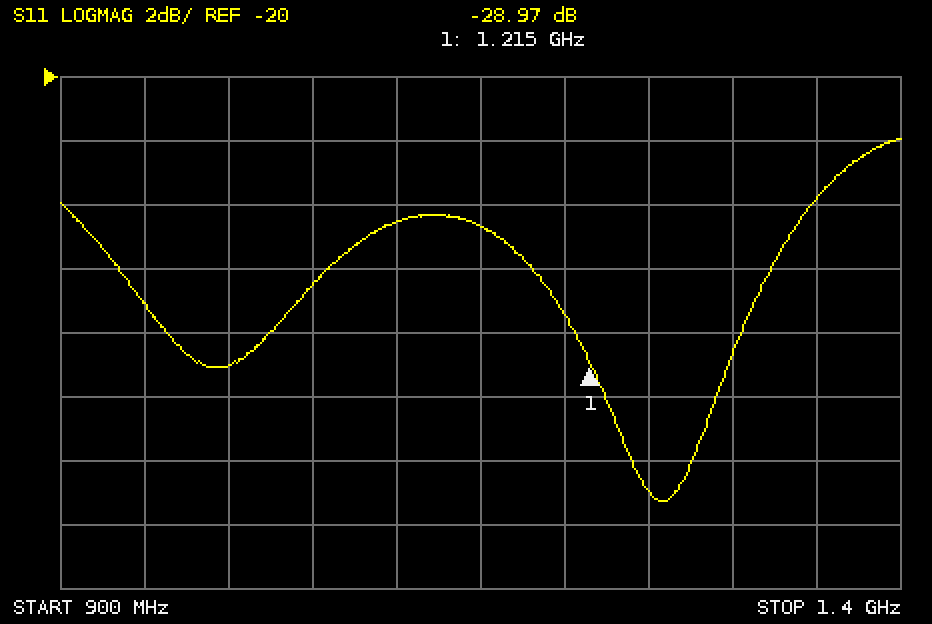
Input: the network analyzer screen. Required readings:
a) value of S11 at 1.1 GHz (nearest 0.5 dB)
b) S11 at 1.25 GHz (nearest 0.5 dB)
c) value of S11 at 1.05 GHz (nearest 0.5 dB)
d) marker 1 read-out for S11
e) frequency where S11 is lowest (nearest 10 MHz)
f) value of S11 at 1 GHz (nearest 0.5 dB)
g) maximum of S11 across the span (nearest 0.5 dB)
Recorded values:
-24.5 dB
-33.0 dB
-26.5 dB
-28.97 dB
1.26 GHz
-29.0 dB
-22.0 dB
